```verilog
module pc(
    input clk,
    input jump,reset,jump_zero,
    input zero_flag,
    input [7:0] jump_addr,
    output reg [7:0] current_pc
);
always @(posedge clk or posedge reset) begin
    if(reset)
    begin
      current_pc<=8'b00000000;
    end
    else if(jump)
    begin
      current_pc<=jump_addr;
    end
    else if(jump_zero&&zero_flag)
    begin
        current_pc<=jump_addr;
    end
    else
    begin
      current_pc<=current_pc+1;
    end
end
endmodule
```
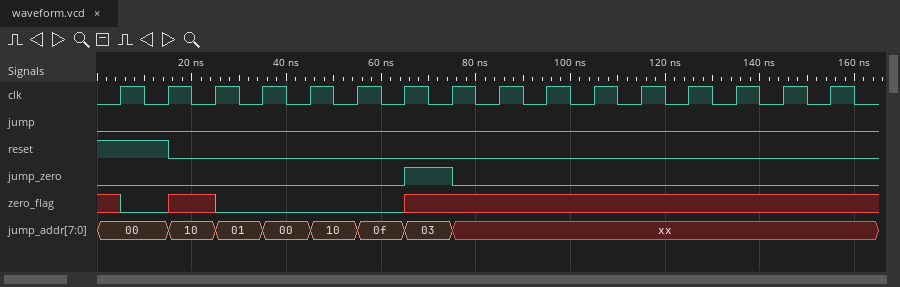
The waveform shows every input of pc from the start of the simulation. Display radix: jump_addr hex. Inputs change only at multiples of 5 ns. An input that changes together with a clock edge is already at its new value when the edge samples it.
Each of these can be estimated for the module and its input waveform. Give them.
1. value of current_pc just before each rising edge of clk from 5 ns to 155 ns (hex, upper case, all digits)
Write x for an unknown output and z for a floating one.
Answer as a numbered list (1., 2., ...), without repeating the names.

1. 00, 00, 01, 02, 03, 04, 05, 06, 07, 08, 09, 0A, 0B, 0C, 0D, 0E
